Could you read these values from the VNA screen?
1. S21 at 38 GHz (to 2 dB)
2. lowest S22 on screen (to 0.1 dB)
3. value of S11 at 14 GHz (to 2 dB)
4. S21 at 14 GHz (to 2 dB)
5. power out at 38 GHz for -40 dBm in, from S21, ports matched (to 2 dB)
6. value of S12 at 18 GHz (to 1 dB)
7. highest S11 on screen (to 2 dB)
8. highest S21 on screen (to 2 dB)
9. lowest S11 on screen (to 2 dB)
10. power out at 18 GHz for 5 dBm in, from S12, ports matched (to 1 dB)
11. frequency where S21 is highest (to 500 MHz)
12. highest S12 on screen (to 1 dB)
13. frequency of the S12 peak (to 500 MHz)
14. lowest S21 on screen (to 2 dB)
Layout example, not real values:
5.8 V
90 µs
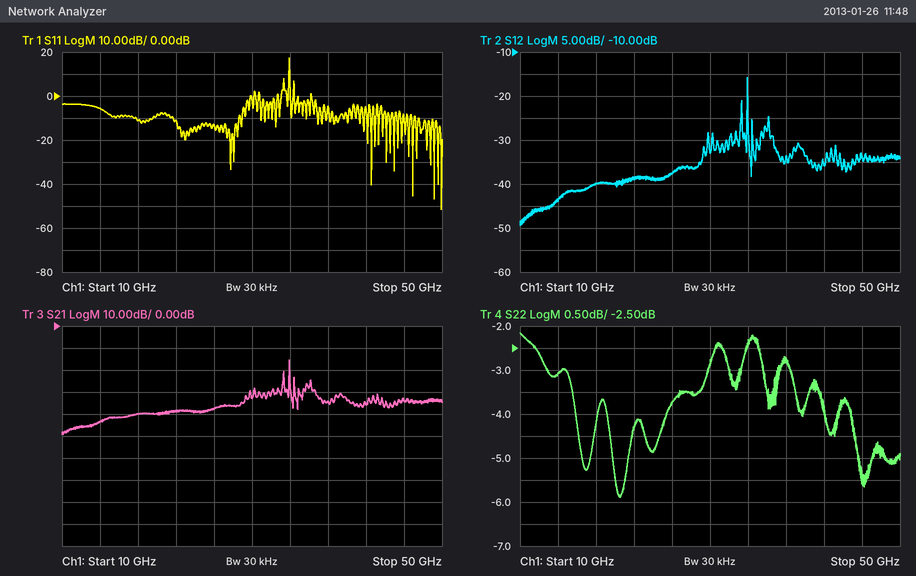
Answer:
-34 dB
-5.9 dB
-6 dB
-44 dB
-74 dBm
-40 dB
18 dB
-16 dB
-52 dB
-35 dBm
34.0 GHz
-16 dB
34.0 GHz
-50 dB
